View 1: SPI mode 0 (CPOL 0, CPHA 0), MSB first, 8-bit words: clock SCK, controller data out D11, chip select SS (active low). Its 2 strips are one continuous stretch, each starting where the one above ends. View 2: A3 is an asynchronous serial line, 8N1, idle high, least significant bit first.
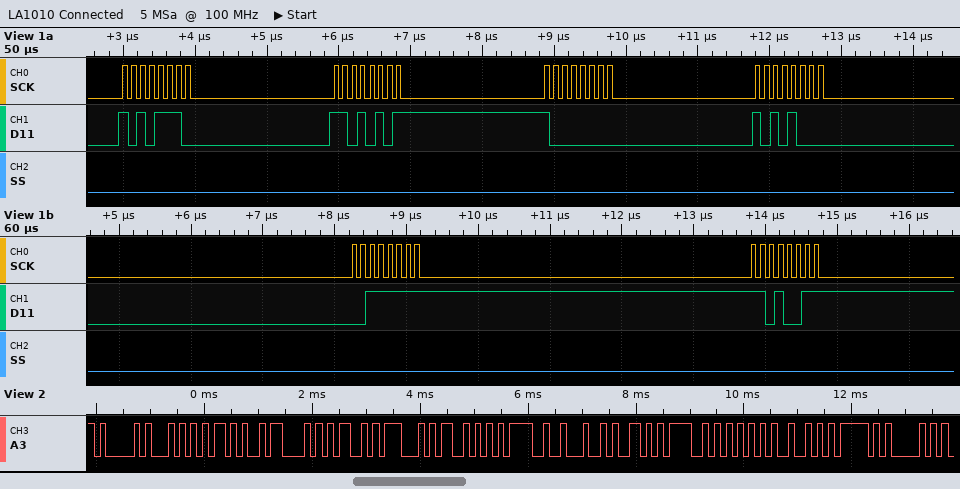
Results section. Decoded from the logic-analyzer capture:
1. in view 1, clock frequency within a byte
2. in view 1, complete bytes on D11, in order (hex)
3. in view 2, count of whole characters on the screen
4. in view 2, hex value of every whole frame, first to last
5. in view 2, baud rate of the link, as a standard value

8 MHz
AE D5 80 A8 3F D3
15
41 54 2B 43 4D 47 53 3D 22 59 4F 55 52 5F 50
9600 baud
